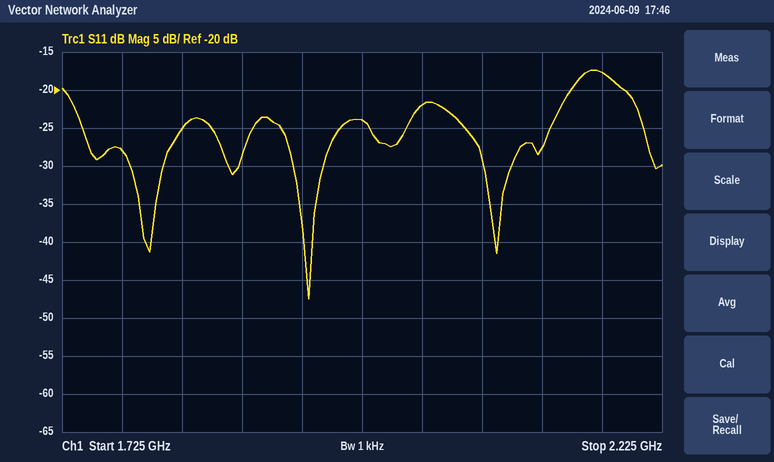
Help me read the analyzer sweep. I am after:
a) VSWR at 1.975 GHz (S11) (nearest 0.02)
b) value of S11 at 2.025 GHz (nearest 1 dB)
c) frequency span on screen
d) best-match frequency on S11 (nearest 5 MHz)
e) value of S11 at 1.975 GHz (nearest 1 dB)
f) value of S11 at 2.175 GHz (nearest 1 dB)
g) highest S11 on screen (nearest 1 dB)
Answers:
1.14
-22 dB
500 MHz
1.930 GHz
-24 dB
-18 dB
-17 dB
